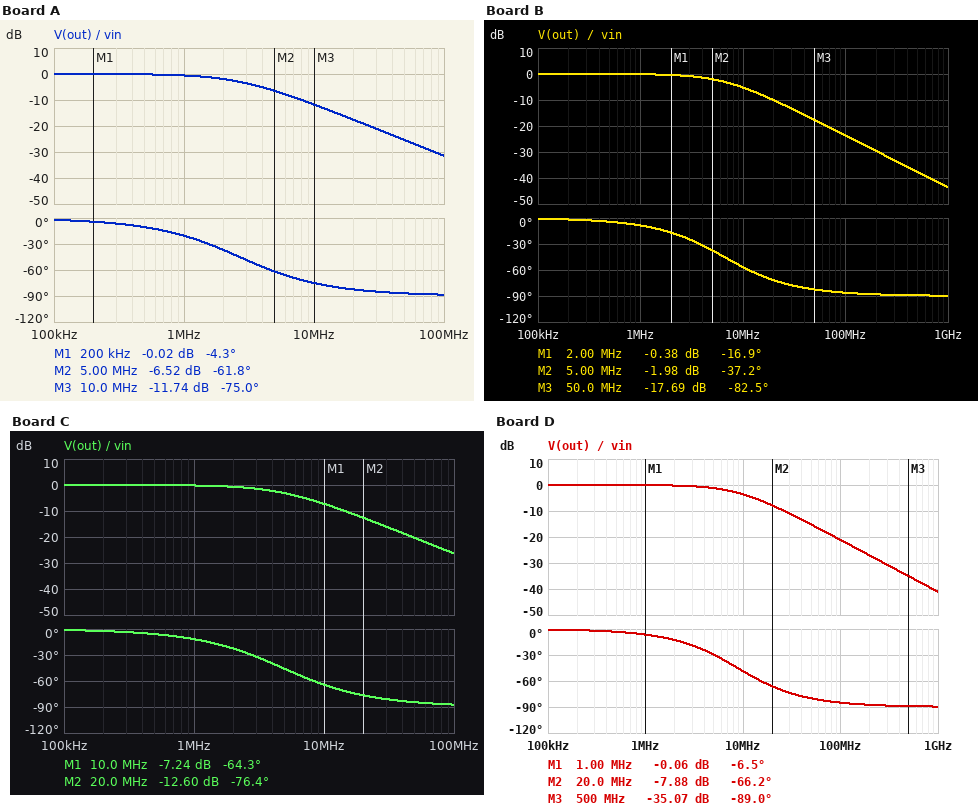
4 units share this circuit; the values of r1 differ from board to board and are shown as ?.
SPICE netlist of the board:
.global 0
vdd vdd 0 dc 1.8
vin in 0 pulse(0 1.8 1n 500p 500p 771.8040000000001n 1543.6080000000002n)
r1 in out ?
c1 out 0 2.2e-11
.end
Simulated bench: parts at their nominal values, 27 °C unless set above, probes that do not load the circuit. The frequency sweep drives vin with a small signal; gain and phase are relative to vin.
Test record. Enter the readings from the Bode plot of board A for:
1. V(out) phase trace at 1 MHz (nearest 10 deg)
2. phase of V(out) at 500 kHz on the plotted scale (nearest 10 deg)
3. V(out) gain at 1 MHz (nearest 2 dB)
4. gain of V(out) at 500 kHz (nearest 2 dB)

-20 deg
-10 deg
0 dB
0 dB
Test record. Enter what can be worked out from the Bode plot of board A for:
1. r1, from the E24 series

2.7 kΩ
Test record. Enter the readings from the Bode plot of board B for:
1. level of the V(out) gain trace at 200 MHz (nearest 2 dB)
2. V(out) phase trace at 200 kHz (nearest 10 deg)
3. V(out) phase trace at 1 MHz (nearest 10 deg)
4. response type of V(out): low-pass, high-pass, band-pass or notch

-30 dB
0 deg
-10 deg
low-pass
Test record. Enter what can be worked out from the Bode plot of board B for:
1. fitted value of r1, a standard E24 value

1.1 kΩ
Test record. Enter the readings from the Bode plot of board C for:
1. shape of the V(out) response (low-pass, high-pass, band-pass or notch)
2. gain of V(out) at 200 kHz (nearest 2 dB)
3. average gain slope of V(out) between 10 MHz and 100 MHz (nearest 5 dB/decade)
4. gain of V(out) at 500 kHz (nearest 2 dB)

low-pass
0 dB
-20 dB/decade
0 dB
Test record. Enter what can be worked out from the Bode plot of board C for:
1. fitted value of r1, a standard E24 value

1.5 kΩ
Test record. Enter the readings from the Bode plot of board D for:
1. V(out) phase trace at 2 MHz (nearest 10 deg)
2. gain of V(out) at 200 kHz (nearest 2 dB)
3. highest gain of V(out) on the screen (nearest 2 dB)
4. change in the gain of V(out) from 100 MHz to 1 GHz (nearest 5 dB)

-10 deg
0 dB
0 dB
-20 dB
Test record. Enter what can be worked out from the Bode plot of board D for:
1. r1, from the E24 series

820 Ω
